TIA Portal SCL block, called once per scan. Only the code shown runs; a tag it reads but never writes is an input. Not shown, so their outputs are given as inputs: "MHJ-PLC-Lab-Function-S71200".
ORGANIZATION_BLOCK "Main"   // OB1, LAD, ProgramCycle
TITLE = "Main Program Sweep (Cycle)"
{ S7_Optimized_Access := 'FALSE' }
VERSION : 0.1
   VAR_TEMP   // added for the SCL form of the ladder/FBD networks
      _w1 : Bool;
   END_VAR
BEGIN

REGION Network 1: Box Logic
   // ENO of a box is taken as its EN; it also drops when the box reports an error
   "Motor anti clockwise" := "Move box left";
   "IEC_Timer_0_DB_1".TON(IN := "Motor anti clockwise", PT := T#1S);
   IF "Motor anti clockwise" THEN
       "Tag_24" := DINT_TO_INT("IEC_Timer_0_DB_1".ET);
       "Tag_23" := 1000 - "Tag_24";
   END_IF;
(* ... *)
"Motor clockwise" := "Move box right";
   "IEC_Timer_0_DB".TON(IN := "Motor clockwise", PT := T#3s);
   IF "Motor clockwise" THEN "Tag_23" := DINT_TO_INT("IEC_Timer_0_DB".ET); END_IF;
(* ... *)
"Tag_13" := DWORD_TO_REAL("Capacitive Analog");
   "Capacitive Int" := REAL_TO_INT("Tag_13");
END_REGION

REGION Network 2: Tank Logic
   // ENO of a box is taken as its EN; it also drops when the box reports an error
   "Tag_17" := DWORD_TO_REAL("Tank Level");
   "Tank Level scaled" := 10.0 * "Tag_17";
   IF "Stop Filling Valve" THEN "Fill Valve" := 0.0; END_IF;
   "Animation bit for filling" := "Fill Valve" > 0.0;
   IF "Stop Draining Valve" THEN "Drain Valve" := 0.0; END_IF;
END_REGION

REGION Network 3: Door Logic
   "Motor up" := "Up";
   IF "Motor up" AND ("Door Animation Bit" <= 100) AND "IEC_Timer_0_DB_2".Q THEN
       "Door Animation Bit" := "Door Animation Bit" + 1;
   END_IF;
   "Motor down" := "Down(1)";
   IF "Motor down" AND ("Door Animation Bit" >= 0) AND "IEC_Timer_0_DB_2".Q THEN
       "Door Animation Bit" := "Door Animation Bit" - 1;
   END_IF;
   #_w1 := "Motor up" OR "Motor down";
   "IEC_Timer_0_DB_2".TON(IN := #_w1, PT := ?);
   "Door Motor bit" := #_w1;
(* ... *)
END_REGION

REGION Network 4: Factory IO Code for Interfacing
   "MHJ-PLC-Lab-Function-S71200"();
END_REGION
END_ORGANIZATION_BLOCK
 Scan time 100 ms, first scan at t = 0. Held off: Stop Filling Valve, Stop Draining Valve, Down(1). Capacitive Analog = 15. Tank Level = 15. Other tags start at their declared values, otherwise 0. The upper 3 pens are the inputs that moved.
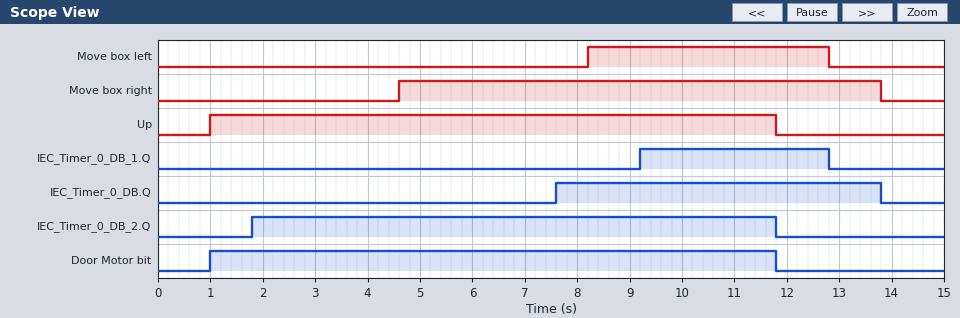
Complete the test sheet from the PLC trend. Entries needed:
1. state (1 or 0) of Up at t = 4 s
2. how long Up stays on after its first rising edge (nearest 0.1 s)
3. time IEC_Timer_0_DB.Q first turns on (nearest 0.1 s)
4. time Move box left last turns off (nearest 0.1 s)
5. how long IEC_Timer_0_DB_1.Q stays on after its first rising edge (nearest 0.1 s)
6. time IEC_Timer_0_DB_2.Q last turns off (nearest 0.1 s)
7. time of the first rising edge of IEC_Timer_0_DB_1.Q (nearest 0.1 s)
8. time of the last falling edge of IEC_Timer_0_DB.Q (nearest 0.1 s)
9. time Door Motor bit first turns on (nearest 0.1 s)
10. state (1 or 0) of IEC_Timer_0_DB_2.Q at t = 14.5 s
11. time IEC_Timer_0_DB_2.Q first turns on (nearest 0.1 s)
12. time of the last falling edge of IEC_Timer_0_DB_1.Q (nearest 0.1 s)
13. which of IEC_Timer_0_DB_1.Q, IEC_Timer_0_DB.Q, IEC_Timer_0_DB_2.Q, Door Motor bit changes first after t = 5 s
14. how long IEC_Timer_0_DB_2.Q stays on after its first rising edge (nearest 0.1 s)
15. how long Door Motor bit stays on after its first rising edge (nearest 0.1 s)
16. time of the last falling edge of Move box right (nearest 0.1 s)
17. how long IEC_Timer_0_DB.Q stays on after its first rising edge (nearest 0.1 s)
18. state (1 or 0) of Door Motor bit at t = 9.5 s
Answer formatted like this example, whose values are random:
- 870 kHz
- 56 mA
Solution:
- 1
- 10.8 s
- 7.6 s
- 12.8 s
- 3.6 s
- 11.8 s
- 9.2 s
- 13.8 s
- 1.0 s
- 0
- 1.8 s
- 12.8 s
- IEC_Timer_0_DB.Q
- 10.0 s
- 10.8 s
- 13.8 s
- 6.2 s
- 1
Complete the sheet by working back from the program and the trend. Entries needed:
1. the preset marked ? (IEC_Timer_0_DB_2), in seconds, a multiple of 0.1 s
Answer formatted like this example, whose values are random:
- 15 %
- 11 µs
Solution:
- 0.8 s
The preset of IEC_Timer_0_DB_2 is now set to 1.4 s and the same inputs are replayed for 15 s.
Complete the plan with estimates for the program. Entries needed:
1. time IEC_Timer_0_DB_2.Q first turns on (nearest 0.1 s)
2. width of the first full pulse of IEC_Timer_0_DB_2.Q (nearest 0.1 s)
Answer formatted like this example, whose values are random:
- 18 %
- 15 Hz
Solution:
- 2.4 s
- 9.4 s
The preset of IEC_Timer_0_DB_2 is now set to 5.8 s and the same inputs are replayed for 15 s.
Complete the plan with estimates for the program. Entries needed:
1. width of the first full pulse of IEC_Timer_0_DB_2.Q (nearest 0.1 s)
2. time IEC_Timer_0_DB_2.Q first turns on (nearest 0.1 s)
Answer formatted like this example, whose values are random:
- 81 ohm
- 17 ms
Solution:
- 5.0 s
- 6.8 s
